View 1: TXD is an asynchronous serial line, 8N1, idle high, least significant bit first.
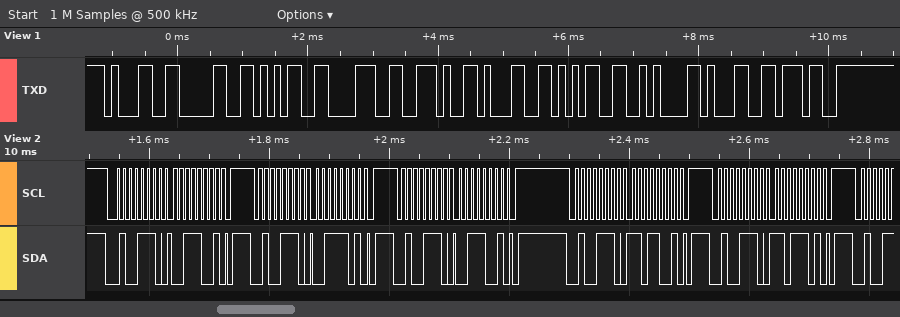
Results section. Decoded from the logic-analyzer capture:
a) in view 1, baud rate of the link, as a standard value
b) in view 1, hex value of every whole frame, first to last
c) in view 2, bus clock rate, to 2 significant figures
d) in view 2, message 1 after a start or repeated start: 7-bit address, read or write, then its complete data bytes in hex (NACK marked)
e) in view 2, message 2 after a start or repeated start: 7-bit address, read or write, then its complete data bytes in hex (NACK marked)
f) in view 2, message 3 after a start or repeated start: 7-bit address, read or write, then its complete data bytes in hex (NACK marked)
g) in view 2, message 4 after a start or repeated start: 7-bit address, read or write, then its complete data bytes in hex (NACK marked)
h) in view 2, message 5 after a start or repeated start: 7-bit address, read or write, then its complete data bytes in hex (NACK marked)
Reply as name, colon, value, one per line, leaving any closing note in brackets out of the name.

in view 1, baud rate of the link, as a standard value: 9600 baud
in view 1, hex value of every whole frame, first to last: 0x31 0x30 0x35 0x38 0x2E 0x31 0x35 0x0A 0x31 0x37
in view 2, bus clock rate, to 2 significant figures: 100 kHz
in view 2, message 1 after a start or repeated start: 7-bit address, read or write, then its complete data bytes in hex: 0x27 write: 39
in view 2, message 2 after a start or repeated start: 7-bit address, read or write, then its complete data bytes in hex: 0x27 write: 3D
in view 2, message 3 after a start or repeated start: 7-bit address, read or write, then its complete data bytes in hex: 0x27 write: 39
in view 2, message 4 after a start or repeated start: 7-bit address, read or write, then its complete data bytes in hex: 0x27 write: D9
in view 2, message 5 after a start or repeated start: 7-bit address, read or write, then its complete data bytes in hex: 0x27 write: DD
